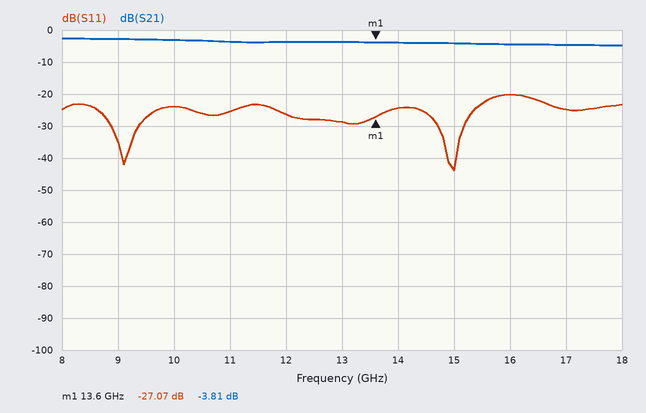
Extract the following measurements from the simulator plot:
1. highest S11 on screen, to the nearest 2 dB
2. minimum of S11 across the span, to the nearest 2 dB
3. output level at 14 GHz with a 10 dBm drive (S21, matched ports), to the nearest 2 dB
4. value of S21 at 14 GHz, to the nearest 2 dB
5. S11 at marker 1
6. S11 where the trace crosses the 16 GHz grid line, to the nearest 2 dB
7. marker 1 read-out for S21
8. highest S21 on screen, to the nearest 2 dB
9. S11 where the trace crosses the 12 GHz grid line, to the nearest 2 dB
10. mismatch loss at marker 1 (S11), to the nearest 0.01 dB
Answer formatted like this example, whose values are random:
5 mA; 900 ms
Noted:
-20 dB; -44 dB; 6 dBm; -4 dB; -27.07 dB; -20 dB; -3.81 dB; -2 dB; -26 dB; 0.01 dB
